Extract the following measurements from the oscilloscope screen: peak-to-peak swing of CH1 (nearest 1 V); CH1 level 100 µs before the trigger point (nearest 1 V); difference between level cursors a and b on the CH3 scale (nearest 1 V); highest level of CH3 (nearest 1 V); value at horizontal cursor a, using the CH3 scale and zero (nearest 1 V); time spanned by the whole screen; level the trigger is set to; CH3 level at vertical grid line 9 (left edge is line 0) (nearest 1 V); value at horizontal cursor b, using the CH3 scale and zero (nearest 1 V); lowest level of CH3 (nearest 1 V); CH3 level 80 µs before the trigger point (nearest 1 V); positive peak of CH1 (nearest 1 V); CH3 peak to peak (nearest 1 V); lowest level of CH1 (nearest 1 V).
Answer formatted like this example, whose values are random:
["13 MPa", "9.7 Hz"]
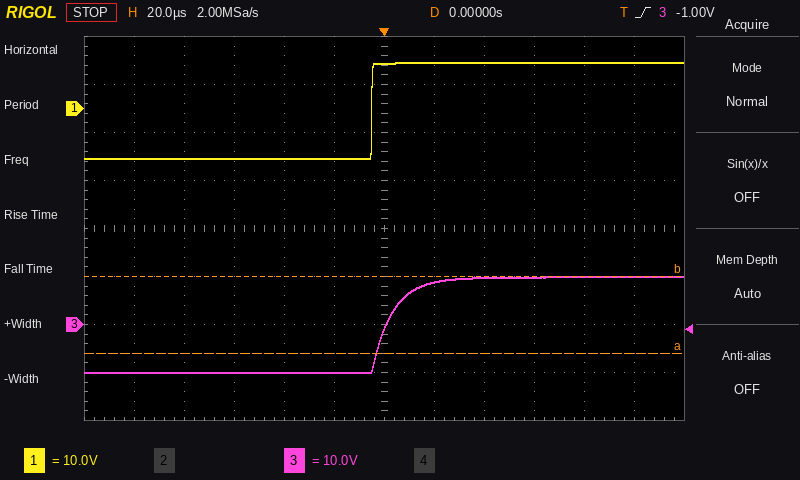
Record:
["20 V", "-10 V", "16 V", "10 V", "-6 V", "240 µs", "-1.00 V", "10 V", "10 V", "-10 V", "-10 V", "10 V", "20 V", "-10 V"]
